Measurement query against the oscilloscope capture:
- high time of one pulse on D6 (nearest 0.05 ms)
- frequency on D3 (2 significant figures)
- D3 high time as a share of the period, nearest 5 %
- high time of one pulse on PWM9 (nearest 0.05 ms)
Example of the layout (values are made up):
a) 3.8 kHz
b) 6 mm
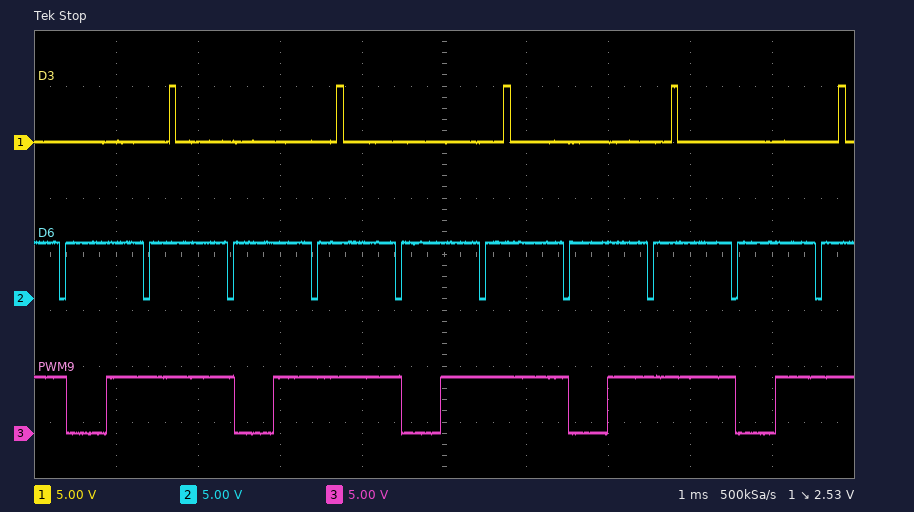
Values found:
a) 0.95 ms
b) 490 Hz
c) 5 %
d) 1.55 ms
